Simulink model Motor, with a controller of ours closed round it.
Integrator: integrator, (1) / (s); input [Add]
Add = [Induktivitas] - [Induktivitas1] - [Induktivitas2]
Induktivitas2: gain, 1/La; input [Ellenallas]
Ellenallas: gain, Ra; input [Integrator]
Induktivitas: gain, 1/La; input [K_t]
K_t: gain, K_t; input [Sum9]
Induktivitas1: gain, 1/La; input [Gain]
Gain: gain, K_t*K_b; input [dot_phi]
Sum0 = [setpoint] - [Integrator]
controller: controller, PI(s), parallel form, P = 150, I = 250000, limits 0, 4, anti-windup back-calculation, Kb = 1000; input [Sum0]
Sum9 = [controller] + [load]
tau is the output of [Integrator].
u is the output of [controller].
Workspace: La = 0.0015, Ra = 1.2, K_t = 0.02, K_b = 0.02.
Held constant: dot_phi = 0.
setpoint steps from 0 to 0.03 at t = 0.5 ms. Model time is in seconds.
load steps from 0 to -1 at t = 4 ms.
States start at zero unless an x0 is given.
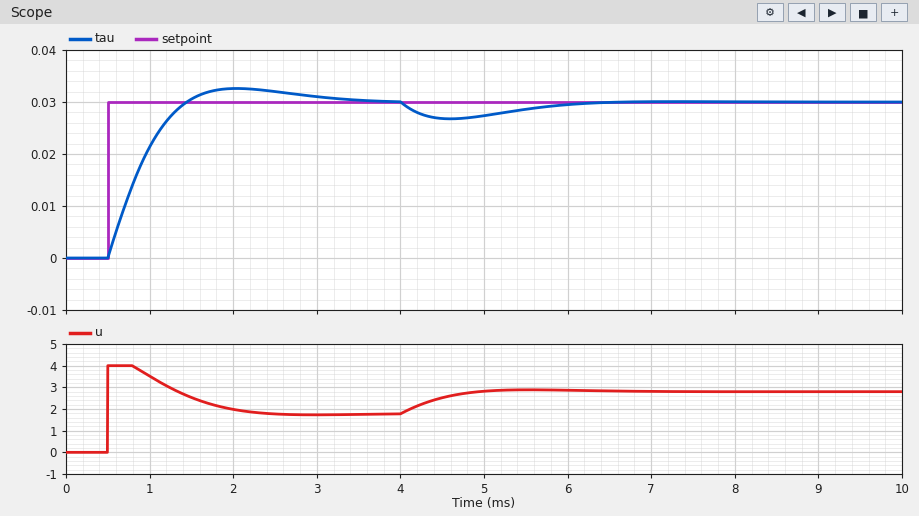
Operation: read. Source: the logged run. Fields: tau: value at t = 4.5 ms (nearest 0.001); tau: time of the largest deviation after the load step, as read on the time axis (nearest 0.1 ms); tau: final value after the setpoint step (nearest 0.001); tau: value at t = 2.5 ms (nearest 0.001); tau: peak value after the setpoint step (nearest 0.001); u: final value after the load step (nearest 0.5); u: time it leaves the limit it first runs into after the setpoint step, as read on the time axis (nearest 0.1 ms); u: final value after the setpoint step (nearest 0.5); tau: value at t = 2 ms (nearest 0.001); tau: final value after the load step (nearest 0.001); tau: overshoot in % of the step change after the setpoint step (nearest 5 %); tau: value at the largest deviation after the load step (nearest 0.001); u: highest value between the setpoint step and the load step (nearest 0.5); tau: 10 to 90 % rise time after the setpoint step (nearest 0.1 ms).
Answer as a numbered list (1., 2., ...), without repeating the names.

1. 0.027
2. 4.6 ms
3. 0.030
4. 0.032
5. 0.033
6. 3.0
7. 0.8 ms
8. 2.0
9. 0.033
10. 0.030
11. 10 %
12. 0.027
13. 4.0
14. 0.7 ms
